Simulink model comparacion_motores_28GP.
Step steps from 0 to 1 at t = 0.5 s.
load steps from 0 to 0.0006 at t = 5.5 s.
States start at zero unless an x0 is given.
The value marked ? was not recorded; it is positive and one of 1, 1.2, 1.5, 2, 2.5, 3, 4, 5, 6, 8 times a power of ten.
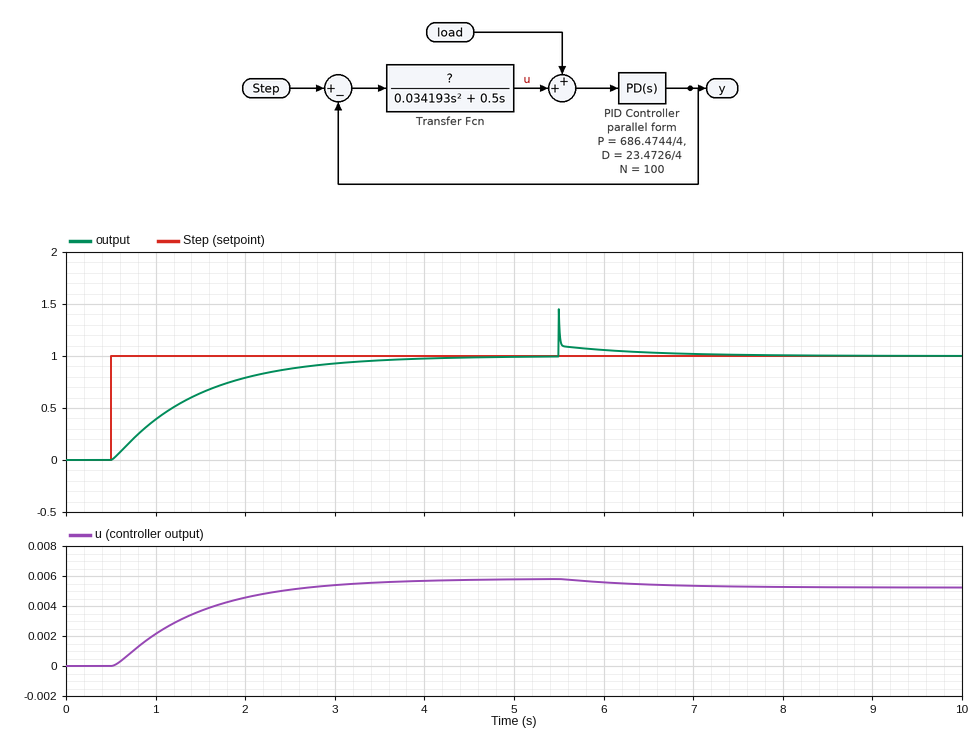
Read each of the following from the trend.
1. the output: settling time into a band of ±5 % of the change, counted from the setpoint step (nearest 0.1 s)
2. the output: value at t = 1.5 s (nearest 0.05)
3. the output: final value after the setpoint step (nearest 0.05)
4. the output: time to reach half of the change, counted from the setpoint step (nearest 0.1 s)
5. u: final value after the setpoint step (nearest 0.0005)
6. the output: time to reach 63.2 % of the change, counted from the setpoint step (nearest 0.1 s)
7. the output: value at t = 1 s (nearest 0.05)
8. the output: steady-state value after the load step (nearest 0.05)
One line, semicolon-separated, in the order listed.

2.8 s; 0.65; 1.00; 0.7 s; 0.0060; 1.0 s; 0.40; 1.00
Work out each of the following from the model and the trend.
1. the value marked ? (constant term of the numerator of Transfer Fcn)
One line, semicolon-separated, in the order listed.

0.003
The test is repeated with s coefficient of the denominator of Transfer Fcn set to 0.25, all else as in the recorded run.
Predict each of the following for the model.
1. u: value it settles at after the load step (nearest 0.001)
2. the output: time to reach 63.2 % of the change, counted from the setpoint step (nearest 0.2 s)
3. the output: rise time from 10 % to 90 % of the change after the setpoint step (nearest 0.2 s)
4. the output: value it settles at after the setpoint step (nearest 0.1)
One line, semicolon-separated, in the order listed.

0.005; 0.6 s; 0.8 s; 1.0
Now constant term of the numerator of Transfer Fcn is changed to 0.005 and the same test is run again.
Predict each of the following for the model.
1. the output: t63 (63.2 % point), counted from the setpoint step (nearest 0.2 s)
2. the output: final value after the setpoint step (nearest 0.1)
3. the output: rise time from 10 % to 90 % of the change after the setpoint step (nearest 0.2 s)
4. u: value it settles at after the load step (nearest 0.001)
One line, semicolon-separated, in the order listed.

0.6 s; 1.0; 1.2 s; 0.005
